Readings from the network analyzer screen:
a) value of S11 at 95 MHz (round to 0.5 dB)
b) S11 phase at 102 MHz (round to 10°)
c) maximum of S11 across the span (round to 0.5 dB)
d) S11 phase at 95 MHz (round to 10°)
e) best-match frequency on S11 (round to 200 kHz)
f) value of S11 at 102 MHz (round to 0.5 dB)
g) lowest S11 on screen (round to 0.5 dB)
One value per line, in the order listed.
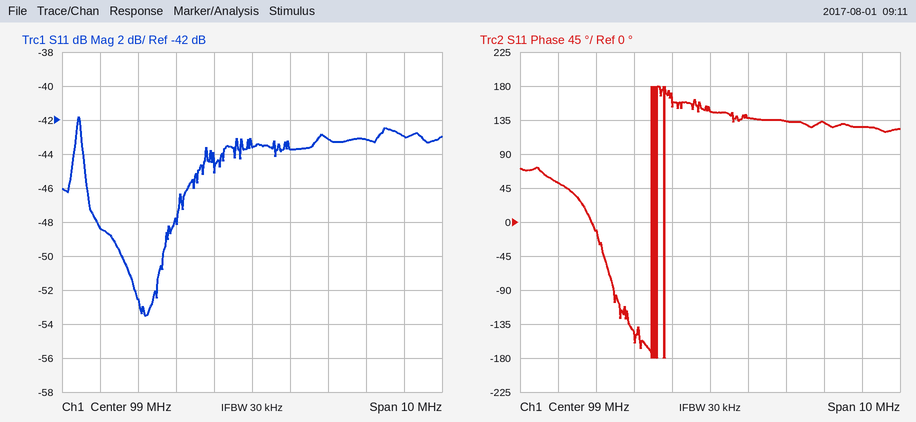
-48.5 dB
130°
-42.0 dB
50°
96.2 MHz
-43.0 dB
-53.5 dB
